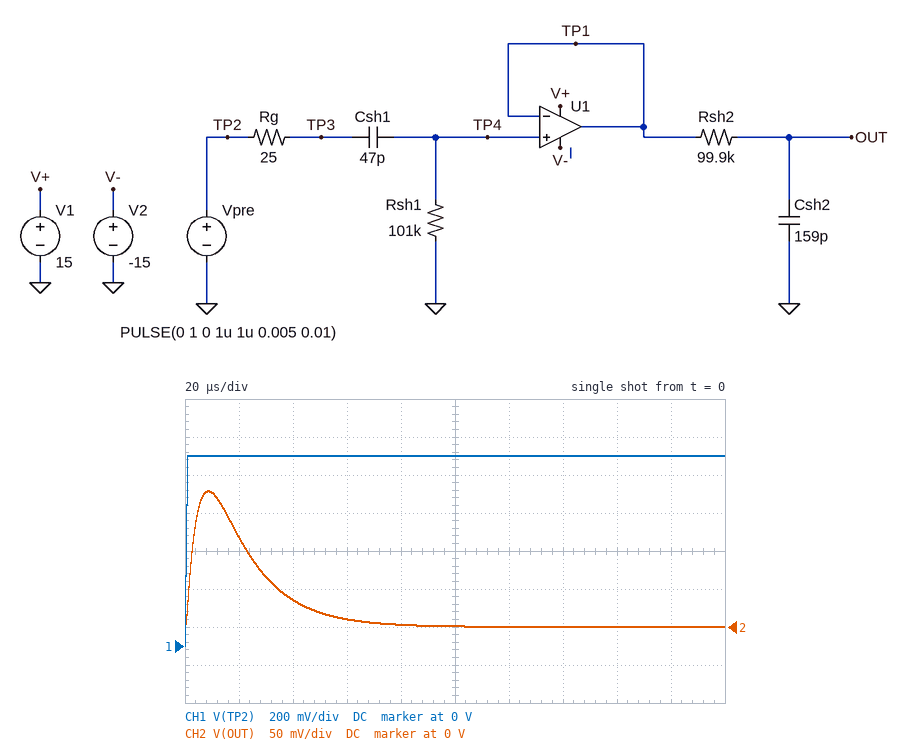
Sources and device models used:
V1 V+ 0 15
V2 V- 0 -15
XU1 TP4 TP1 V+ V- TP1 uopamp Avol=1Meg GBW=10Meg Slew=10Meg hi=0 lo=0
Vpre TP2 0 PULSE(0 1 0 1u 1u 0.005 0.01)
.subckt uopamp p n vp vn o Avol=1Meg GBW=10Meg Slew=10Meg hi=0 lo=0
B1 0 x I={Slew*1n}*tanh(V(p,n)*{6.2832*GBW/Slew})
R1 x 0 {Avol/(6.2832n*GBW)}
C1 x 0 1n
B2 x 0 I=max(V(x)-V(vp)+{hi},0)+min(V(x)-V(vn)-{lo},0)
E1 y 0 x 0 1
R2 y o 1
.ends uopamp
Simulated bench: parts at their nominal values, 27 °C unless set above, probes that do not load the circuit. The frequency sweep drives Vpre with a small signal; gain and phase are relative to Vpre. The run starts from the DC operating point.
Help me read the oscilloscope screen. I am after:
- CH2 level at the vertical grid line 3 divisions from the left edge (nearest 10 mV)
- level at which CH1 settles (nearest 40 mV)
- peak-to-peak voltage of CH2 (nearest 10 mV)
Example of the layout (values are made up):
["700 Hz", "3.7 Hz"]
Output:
["10 mV", "1.00 V", "180 mV"]
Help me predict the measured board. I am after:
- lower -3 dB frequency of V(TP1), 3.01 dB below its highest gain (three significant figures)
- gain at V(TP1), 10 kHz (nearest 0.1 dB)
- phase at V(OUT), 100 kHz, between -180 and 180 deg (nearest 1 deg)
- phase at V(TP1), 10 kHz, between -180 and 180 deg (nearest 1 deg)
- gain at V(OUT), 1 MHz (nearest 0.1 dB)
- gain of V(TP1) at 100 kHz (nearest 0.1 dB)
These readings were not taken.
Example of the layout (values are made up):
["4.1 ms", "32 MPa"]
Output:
["33.3 kHz", "-10.9 dB", "-66 deg", "73 deg", "-40.0 dB", "-0.5 dB"]
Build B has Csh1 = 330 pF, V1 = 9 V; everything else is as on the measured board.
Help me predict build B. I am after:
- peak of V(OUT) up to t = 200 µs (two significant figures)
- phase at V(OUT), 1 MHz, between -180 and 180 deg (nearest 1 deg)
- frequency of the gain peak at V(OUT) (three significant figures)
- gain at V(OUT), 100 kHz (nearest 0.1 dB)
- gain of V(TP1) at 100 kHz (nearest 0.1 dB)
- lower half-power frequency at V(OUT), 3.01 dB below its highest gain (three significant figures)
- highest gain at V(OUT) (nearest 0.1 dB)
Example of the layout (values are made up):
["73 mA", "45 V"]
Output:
["510 mV", "-95 deg", "6.92 kHz", "-20.0 dB", "0 dB", "2.73 kHz", "-3.4 dB"]
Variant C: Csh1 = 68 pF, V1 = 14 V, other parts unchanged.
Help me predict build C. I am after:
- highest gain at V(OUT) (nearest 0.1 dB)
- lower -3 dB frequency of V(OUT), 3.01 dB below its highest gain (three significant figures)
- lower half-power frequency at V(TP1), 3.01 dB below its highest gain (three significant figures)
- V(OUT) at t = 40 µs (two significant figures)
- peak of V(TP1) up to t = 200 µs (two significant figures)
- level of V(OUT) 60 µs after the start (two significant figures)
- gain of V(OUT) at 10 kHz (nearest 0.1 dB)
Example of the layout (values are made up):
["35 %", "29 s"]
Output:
["-10.4 dB", "5.93 kHz", "23.1 kHz", "61 mV", "930 mV", "18 mV", "-11.0 dB"]
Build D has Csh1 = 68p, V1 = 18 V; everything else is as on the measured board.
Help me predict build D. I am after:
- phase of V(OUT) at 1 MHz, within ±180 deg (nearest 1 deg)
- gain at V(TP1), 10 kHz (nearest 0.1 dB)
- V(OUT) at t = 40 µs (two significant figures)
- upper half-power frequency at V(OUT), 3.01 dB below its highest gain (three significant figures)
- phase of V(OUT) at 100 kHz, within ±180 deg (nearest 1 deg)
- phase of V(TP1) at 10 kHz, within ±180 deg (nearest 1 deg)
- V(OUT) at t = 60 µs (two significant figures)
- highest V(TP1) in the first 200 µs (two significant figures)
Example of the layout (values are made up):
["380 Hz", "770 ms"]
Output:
["-94 deg", "-8.0 dB", "61 mV", "39.1 kHz", "-72 deg", "67 deg", "18 mV", "930 mV"]
